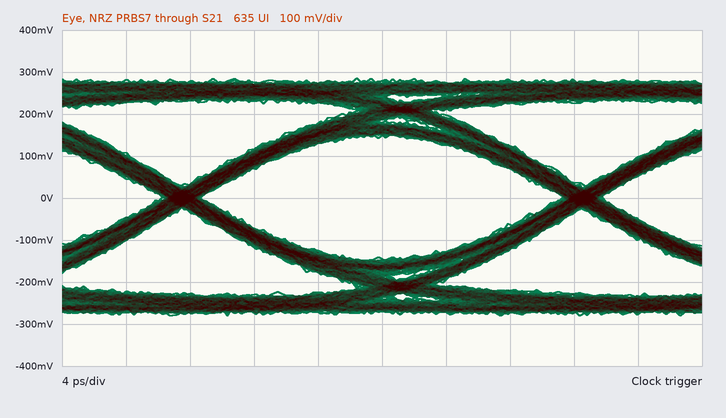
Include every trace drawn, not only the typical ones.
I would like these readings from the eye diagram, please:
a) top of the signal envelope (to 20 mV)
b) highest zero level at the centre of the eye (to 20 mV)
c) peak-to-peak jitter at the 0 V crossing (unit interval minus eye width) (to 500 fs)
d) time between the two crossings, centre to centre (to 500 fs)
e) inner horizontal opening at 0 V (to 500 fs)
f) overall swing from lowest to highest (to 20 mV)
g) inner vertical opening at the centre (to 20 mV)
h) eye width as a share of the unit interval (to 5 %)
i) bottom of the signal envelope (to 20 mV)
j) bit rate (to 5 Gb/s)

280 mV
-140 mV
2.5 ps
25.0 ps
22.5 ps
560 mV
300 mV
90 %
-280 mV
40 Gb/s
